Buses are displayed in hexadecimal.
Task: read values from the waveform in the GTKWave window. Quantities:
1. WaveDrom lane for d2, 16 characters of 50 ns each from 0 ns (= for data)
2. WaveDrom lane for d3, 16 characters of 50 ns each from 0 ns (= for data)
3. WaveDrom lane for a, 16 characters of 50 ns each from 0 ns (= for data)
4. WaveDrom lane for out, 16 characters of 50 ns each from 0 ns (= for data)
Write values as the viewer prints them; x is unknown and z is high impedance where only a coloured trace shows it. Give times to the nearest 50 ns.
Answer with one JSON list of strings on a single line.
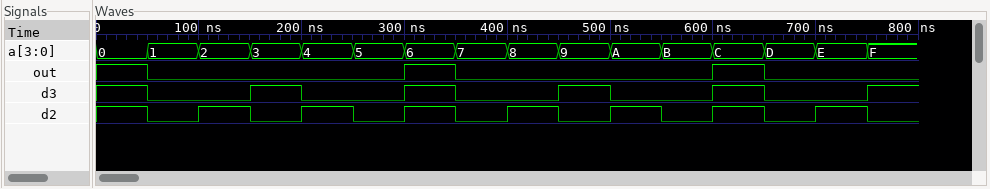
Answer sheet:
["{name: 'd2', wave: '1010101010101010'}", "{name: 'd3', wave: '10.10.10.10.10.1'}", "{name: 'a', wave: '================', data: '0 1 2 3 4 5 6 7 8 9 A B C D E F'}", "{name: 'out', wave: '10....10....10..'}"]
